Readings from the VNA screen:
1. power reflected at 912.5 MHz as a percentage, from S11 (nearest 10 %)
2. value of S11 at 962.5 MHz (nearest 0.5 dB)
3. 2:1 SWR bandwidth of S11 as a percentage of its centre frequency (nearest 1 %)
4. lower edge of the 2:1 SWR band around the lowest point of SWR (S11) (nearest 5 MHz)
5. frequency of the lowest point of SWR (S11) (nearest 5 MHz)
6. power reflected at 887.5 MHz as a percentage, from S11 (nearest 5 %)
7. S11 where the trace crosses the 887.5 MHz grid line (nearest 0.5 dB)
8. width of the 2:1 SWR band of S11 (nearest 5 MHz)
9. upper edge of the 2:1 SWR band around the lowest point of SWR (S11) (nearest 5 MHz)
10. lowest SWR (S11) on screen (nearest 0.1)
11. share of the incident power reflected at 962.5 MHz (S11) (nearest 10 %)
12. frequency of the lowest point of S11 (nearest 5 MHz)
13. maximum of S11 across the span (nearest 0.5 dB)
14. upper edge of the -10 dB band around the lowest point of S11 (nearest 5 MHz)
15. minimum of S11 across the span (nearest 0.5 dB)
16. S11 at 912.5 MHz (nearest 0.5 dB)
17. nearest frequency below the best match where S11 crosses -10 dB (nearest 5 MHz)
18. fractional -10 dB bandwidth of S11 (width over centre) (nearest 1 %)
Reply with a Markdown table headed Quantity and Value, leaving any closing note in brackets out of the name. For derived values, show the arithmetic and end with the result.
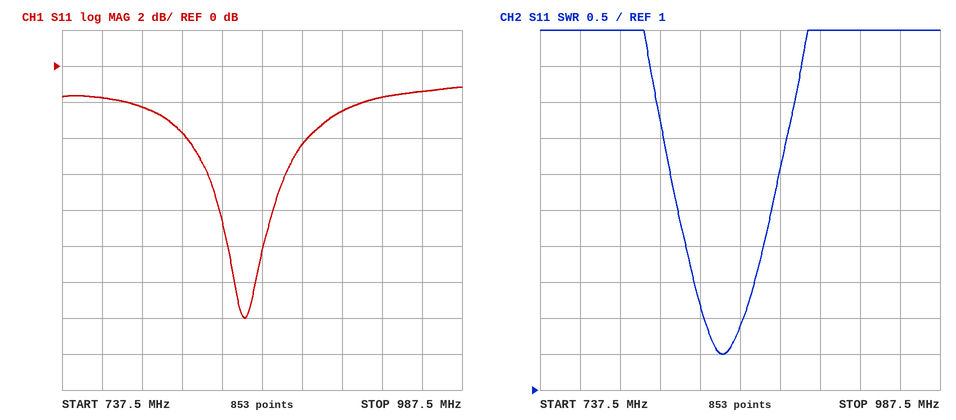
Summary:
| Quantity | Value |
|---|---|
| power reflected at 912.5 MHz as a percentage, from S11 | 10^(-2.5/10) ≈ 56.2 %, so 60 % to the nearest 10 % |
| value of S11 at 962.5 MHz | -1.5 dB |
| 2:1 SWR bandwidth of S11 as a percentage of its centre frequency | 25 MHz / 852.5 MHz ≈ 3 % |
| lower edge of the 2:1 SWR band around the lowest point of SWR (S11) | 840 MHz |
| frequency of the lowest point of SWR (S11) | 850 MHz |
| power reflected at 887.5 MHz as a percentage, from S11 | 10^(-4.5/10) ≈ 35 % |
| S11 where the trace crosses the 887.5 MHz grid line | -4.5 dB |
| width of the 2:1 SWR band of S11 | 865 MHz − 840 MHz = 25 MHz |
| upper edge of the 2:1 SWR band around the lowest point of SWR (S11) | 865 MHz |
| lowest SWR (S11) on screen | 1.5 |
| share of the incident power reflected at 962.5 MHz (S11) | 10^(-1.5/10) ≈ 70.8 %, so 70 % to the nearest 10 % |
| frequency of the lowest point of S11 | 850 MHz |
| maximum of S11 across the span | -1.0 dB |
| upper edge of the -10 dB band around the lowest point of S11 | 865 MHz |
| minimum of S11 across the span | -14.0 dB |
| S11 at 912.5 MHz | -2.5 dB |
| nearest frequency below the best match where S11 crosses -10 dB | 840 MHz |
| fractional -10 dB bandwidth of S11 (width over centre) | 25 MHz / 852.5 MHz ≈ 3 % |
